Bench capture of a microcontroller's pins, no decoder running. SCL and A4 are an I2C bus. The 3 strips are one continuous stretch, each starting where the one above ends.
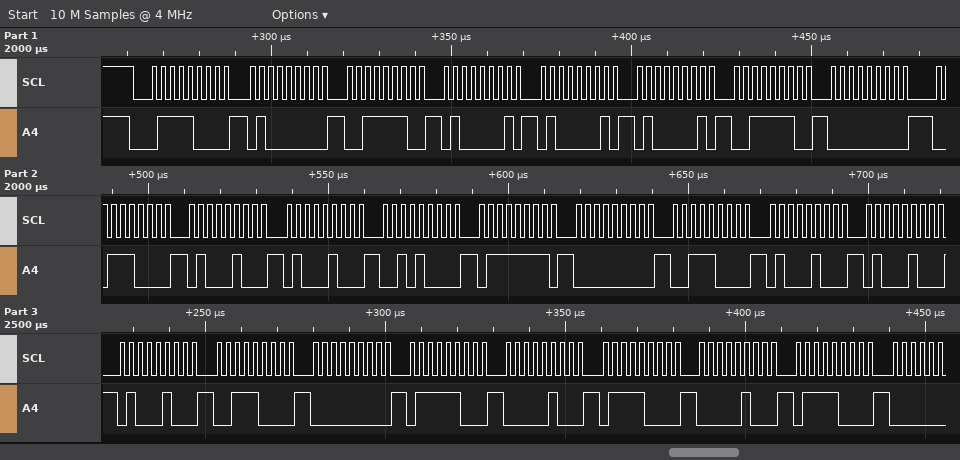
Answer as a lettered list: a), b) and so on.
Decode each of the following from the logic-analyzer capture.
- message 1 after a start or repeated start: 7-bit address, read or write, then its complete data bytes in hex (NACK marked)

a) 0x3C write: 40 3E 41 41 41 3E 00 38 44 44 28 7F 00 38 44 44 44 38 00 7C 04 78 04 78
